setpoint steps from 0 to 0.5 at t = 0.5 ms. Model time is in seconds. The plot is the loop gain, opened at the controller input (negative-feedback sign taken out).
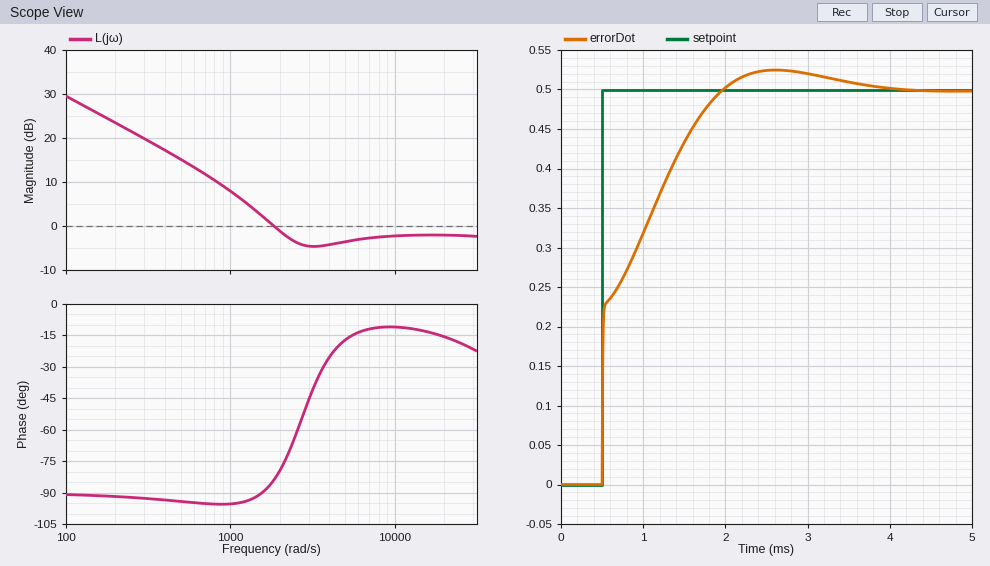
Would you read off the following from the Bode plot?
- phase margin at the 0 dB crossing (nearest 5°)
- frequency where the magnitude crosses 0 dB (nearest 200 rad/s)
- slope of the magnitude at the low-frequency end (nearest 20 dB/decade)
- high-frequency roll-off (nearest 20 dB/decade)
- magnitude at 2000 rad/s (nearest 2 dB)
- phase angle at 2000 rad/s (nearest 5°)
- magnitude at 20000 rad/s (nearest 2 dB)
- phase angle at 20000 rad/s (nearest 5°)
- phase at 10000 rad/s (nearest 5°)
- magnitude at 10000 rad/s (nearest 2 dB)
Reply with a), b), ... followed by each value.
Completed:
a) 95°
b) 1800 rad/s
c) -20 dB/decade
d) 0 dB/decade
e) -2 dB
f) -80°
g) -2 dB
h) -15°
i) -10°
j) -2 dB
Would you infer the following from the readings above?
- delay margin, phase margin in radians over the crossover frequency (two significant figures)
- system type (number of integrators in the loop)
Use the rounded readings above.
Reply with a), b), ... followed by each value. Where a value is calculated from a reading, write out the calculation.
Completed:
a) 95 × π / 180 / 1800 = 0.00092 s
b) 1
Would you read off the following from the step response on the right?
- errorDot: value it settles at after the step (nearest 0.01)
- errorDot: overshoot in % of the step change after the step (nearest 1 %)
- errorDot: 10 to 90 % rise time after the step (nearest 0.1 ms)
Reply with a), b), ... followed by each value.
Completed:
a) 0.50
b) 5 %
c) 1.1 ms
